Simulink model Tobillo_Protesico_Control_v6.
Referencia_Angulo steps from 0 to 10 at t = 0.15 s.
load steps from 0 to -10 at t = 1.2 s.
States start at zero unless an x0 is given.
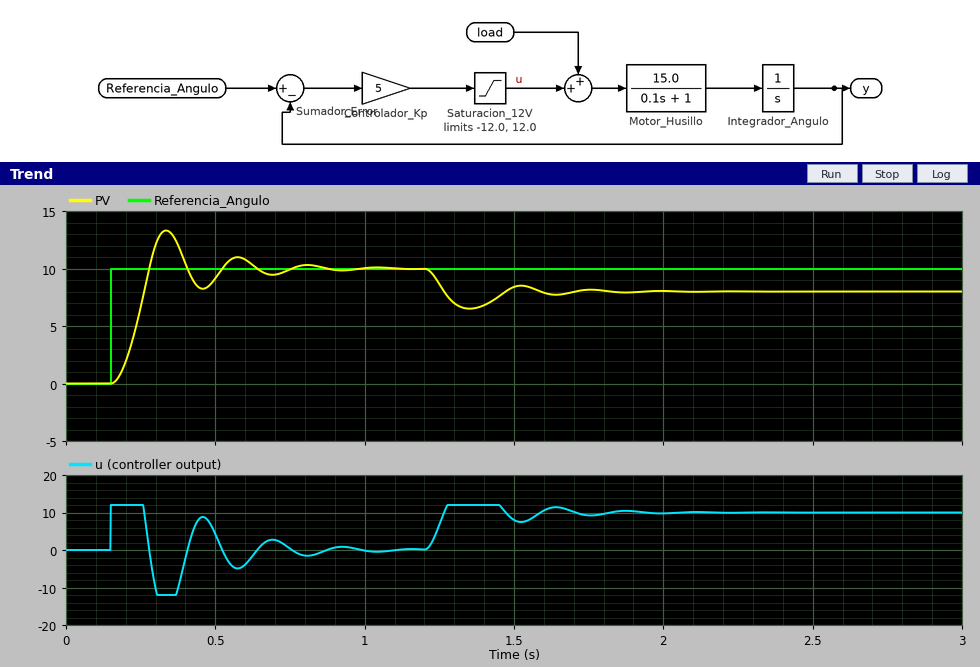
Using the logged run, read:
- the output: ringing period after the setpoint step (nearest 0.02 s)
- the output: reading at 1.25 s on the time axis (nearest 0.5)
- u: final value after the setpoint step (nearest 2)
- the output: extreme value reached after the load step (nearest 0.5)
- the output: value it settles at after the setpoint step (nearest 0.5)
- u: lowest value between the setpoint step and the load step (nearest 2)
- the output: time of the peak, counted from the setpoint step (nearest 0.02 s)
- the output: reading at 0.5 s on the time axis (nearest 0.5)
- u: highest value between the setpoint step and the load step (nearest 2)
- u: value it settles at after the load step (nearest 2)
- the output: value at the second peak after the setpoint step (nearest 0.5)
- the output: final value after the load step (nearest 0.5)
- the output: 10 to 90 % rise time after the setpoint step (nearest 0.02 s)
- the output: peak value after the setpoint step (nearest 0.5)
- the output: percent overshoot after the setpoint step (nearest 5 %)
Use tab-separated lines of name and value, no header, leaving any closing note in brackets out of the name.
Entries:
the output: ringing period after the setpoint step	0.24 s
the output: reading at 1.25 s on the time axis	8.5
u: final value after the setpoint step	0
the output: extreme value reached after the load step	6.5
the output: value it settles at after the setpoint step	10.0
u: lowest value between the setpoint step and the load step	-12
the output: time of the peak, counted from the setpoint step	0.18 s
the output: reading at 0.5 s on the time axis	9.0
u: highest value between the setpoint step and the load step	12
u: value it settles at after the load step	10
the output: value at the second peak after the setpoint step	11.0
the output: final value after the load step	8.0
the output: 10 to 90 % rise time after the setpoint step	0.08 s
the output: peak value after the setpoint step	13.5
the output: percent overshoot after the setpoint step	35 %
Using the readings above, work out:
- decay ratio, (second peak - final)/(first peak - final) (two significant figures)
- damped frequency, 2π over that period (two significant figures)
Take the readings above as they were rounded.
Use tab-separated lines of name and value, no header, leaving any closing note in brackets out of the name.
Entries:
decay ratio, (second peak - final)/(first peak - final)	0.29
damped frequency, 2π over that period	26 rad/s
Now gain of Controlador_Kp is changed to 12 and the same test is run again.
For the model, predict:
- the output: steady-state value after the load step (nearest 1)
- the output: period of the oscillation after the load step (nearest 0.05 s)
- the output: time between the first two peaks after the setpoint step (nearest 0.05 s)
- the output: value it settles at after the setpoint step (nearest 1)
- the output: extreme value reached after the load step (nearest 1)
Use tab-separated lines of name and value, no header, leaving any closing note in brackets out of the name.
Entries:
the output: steady-state value after the load step	9
the output: period of the oscillation after the load step	0.20 s
the output: time between the first two peaks after the setpoint step	0.20 s
the output: value it settles at after the setpoint step	10
the output: extreme value reached after the load step	8
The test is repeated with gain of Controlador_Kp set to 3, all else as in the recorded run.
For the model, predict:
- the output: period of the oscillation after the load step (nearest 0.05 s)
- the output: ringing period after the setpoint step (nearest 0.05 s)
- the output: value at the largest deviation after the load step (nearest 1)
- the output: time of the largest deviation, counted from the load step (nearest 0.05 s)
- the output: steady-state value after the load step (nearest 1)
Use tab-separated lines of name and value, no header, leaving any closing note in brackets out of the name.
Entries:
the output: period of the oscillation after the load step	0.35 s
the output: ringing period after the setpoint step	0.30 s
the output: value at the largest deviation after the load step	5
the output: time of the largest deviation, counted from the load step	0.20 s
the output: steady-state value after the load step	7
